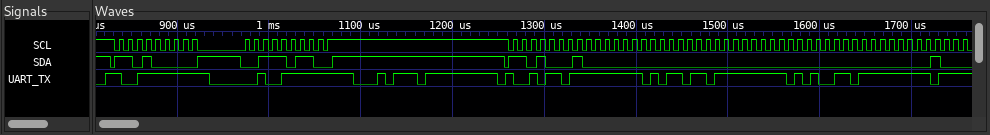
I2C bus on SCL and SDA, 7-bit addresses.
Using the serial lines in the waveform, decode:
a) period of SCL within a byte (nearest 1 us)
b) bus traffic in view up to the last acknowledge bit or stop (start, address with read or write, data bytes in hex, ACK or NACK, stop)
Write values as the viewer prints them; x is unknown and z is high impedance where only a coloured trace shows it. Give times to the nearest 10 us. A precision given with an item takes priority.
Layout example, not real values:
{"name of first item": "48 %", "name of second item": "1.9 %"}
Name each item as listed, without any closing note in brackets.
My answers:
{"period of SCL within a byte": "10 us", "bus traffic in view up to the last acknowledge bit or stop": "start, address 68 write ACK, 3B ACK, stop, start, address 68 read ACK, 00 ACK, 00 ACK, 00 ACK, 00 ACK"}
